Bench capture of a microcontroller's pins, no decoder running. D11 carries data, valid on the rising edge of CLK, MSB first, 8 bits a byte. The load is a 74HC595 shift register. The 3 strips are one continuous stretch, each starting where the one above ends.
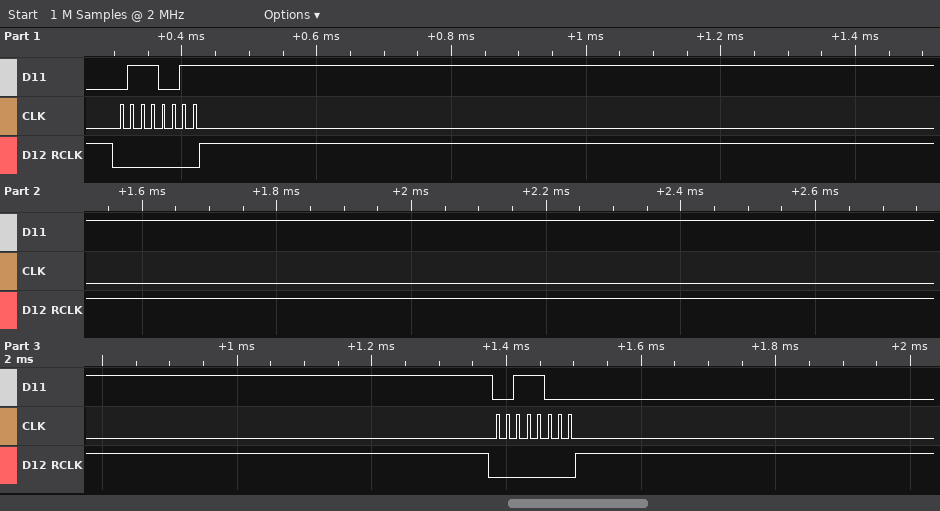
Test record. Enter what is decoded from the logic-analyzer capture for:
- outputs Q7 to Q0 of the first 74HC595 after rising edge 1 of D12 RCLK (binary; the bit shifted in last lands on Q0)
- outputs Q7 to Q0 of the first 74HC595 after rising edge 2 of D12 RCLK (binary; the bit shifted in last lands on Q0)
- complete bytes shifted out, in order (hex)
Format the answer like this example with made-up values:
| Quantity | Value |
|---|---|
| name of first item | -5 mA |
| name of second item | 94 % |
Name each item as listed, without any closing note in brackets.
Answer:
| Quantity | Value |
|---|---|
| outputs Q7 to Q0 of the first 74HC595 after rising edge 1 of D12 RCLK | 01110011 |
| outputs Q7 to Q0 of the first 74HC595 after rising edge 2 of D12 RCLK | 00111000 |
| complete bytes shifted out, in order | 0x73 0x38 |
